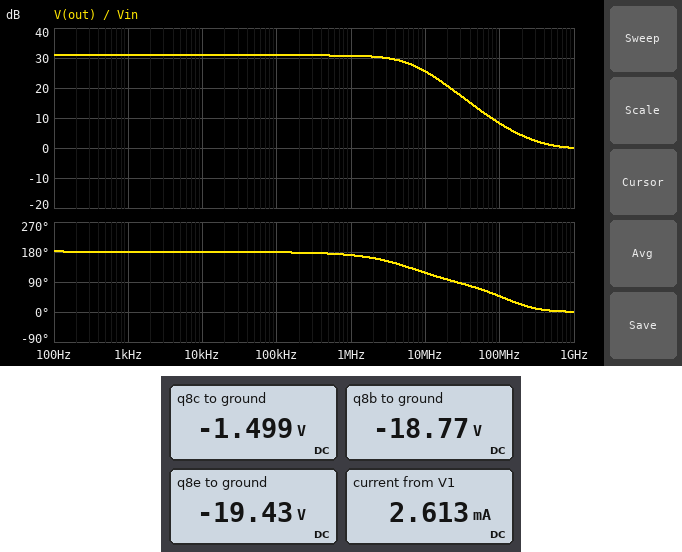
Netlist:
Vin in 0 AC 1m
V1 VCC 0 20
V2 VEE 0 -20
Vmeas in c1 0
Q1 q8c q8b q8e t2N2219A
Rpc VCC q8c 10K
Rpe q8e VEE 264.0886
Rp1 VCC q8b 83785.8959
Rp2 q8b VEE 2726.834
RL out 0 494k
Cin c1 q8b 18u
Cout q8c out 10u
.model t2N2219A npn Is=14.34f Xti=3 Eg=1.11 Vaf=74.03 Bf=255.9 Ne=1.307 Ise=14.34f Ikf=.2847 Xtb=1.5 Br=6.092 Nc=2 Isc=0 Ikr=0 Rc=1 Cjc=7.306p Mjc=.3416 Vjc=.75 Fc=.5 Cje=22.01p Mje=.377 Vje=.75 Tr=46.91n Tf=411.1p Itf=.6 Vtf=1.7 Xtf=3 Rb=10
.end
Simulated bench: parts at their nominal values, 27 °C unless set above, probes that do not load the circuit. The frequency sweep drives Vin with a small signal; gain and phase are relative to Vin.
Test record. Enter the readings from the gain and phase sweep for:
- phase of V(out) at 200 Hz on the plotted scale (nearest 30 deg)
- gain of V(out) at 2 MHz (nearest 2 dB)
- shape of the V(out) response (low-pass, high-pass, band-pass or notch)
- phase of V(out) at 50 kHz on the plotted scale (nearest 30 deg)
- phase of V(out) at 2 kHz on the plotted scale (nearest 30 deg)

180 deg
30 dB
low-pass
180 deg
180 deg
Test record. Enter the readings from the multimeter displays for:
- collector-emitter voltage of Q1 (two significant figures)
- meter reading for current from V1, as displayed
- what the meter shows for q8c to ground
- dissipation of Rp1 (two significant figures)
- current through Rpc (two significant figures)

18 V
2.613 mA
-1.499 V
18 mW
2.1 mA
